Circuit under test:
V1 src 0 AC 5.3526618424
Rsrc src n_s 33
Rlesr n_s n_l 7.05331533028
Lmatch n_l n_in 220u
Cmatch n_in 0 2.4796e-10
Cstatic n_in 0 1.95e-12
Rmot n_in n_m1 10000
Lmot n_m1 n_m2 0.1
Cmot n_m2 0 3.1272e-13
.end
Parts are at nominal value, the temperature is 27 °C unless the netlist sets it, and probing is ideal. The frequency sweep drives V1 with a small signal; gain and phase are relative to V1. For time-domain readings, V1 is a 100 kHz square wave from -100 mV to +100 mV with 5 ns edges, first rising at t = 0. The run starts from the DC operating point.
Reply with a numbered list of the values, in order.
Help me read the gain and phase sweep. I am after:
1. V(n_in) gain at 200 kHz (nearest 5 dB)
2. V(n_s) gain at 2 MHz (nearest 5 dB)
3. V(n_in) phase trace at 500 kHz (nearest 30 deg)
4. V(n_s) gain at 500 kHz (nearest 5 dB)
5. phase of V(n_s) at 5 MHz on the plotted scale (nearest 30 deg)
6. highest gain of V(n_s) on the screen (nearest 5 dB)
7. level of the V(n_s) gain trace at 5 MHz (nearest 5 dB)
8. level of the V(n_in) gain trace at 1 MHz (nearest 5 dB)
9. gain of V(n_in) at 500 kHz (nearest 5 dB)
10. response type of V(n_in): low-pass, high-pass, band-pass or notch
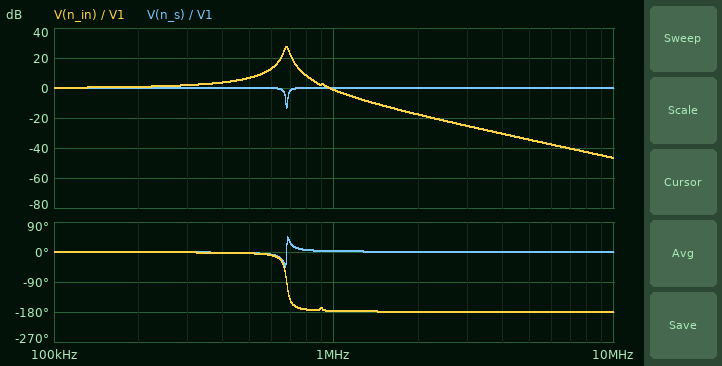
1. 0 dB
2. 0 dB
3. 0 deg
4. 0 dB
5. 0 deg
6. 0 dB
7. 0 dB
8. 0 dB
9. 5 dB
10. low-pass
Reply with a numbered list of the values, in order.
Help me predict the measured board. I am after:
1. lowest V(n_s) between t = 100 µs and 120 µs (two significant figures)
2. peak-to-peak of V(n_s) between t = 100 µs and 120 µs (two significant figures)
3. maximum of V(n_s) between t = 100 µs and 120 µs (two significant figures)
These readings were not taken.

1. -110 mV
2. 220 mV
3. 110 mV
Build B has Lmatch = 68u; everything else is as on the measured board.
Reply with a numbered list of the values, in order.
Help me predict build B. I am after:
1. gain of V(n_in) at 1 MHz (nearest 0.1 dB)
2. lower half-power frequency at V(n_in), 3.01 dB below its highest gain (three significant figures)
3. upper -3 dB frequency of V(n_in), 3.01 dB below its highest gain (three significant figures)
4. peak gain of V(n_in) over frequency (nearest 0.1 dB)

1. 9.4 dB
2. 1.17 MHz
3. 1.27 MHz
4. 22.3 dB
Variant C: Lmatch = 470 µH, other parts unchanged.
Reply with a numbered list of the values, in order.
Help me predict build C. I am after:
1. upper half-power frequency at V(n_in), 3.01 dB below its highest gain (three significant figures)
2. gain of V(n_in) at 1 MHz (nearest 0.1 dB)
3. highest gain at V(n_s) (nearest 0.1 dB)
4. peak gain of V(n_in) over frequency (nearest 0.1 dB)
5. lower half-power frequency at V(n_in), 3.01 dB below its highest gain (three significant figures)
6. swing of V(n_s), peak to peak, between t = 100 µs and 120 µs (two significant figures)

1. 471 kHz
2. -11.2 dB
3. 0 dB
4. 30.7 dB
5. 457 kHz
6. 210 mV
